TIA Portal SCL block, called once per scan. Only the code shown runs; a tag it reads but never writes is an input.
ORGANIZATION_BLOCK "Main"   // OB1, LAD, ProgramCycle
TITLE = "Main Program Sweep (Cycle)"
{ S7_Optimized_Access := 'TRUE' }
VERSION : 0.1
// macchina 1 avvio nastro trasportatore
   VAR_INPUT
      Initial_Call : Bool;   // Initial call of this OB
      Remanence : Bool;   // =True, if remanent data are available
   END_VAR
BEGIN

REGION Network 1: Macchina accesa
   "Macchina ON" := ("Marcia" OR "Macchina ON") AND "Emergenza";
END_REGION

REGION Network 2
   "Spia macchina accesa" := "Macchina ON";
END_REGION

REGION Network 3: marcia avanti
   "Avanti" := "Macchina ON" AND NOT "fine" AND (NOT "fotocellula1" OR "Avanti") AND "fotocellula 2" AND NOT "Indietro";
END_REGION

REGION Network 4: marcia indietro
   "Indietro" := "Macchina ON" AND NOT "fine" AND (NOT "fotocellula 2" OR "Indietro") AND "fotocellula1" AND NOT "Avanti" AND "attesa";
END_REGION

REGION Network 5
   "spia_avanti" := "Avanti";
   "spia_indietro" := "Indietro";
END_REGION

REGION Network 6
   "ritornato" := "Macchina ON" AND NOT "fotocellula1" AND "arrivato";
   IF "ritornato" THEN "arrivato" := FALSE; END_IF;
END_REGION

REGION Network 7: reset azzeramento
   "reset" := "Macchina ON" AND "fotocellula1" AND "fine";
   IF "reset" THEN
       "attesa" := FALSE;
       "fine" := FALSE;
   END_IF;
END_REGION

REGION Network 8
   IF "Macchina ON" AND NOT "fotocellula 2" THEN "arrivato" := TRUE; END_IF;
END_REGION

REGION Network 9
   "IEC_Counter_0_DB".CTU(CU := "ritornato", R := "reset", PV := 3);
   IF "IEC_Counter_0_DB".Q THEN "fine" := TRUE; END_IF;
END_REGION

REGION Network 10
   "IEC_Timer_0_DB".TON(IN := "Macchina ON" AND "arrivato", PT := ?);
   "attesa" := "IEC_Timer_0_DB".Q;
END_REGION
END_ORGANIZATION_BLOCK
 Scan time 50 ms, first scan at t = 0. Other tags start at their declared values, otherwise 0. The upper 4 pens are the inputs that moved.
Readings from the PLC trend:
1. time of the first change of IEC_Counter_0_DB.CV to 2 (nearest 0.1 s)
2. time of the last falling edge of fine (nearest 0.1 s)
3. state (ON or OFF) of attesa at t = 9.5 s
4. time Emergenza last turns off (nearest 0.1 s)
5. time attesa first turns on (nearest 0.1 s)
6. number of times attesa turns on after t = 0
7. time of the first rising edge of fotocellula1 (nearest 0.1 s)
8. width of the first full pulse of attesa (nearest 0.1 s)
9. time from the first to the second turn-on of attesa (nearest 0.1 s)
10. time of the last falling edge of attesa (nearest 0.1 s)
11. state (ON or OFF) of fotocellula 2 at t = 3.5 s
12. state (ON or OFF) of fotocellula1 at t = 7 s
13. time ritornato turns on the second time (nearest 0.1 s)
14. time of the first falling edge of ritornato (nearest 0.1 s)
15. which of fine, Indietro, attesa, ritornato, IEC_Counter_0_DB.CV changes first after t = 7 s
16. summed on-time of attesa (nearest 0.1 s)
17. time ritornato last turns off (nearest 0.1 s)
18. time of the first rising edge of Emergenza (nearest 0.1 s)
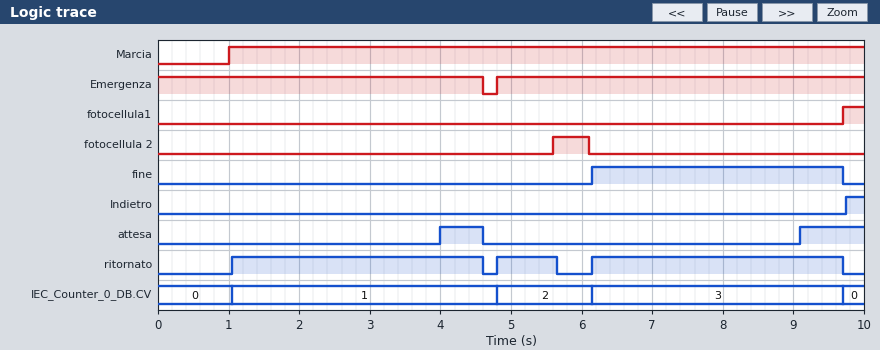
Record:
4.8 s
9.7 s
ON
4.6 s
4.0 s
2
9.7 s
0.6 s
5.1 s
4.6 s
OFF
OFF
4.8 s
4.6 s
attesa
1.5 s
9.7 s
4.8 s
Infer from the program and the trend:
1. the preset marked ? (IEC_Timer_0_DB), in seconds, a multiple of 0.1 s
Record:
3.0 s
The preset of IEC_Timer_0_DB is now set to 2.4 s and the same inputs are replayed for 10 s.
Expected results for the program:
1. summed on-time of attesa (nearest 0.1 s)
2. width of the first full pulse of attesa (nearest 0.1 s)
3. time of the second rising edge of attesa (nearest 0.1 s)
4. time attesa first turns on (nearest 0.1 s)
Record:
2.7 s
1.2 s
8.5 s
3.4 s
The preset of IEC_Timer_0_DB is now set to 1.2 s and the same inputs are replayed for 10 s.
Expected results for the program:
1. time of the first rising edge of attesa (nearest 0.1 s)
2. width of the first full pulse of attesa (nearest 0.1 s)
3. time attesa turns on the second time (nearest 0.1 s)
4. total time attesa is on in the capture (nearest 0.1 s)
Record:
2.2 s
2.4 s
7.3 s
5.1 s
